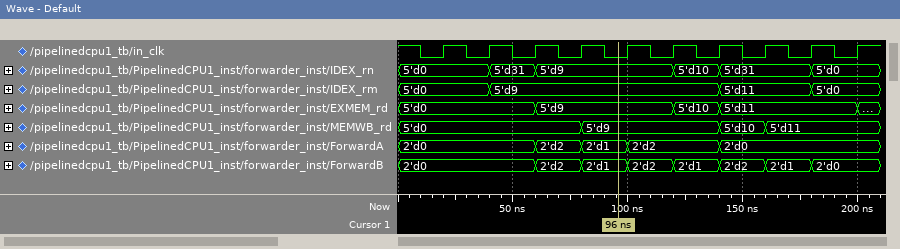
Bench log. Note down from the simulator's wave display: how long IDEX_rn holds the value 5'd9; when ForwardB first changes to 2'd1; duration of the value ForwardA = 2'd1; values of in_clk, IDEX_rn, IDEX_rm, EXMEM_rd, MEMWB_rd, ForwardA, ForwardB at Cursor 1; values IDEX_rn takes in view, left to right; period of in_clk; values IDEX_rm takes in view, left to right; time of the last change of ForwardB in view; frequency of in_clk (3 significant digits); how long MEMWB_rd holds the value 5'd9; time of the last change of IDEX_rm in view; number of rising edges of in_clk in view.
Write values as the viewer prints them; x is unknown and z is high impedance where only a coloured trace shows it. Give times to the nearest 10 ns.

60 ns
80 ns
20 ns
in_clk=0, IDEX_rn=5'd9, IDEX_rm=5'd9, EXMEM_rd=5'd9, MEMWB_rd=5'd9, ForwardA=2'd1, ForwardB=2'd1
5'd0, 5'd31, 5'd9, 5'd10, 5'd31, 5'd0
20 ns
5'd0, 5'd9, 5'd11, 5'd0
180 ns
50.0 MHz
60 ns
180 ns
10
